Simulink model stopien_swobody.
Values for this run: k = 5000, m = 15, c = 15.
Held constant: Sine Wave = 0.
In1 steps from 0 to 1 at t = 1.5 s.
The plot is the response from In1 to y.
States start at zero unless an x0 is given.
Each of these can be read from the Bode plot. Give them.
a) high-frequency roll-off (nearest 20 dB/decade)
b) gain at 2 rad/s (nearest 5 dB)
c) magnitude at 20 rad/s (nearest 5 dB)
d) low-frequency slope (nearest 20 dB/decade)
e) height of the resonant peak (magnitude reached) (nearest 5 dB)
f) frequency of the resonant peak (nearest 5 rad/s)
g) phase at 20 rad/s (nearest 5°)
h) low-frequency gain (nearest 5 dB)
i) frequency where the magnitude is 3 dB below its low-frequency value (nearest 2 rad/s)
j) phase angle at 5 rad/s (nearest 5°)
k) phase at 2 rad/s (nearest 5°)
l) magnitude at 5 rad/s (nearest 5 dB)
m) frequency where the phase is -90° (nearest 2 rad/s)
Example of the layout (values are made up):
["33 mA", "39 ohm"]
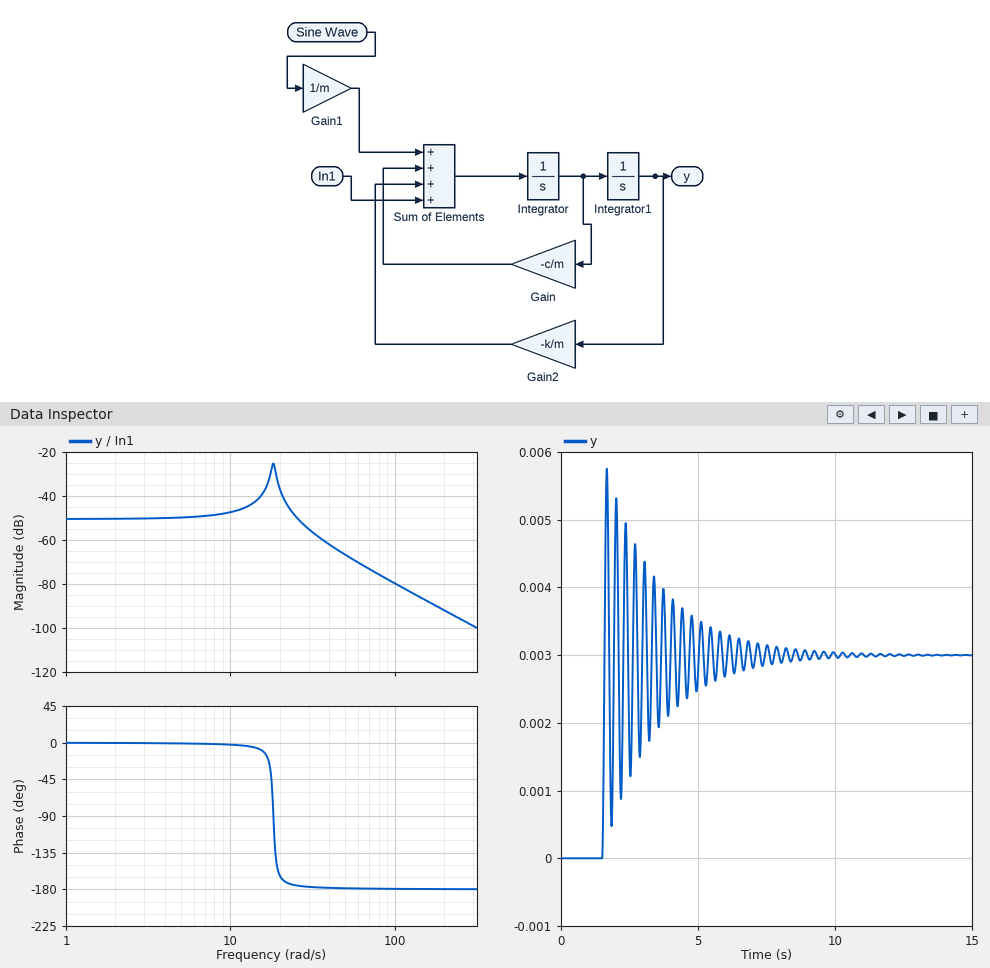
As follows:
["-40 dB/decade", "-50 dB", "-35 dB", "0 dB/decade", "-25 dB", "20 rad/s", "-165°", "-50 dB", "28 rad/s", "0°", "0°", "-50 dB", "18 rad/s"]
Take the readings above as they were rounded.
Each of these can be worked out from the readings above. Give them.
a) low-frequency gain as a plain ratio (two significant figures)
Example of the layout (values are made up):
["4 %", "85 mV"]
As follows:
["0.0032"]
